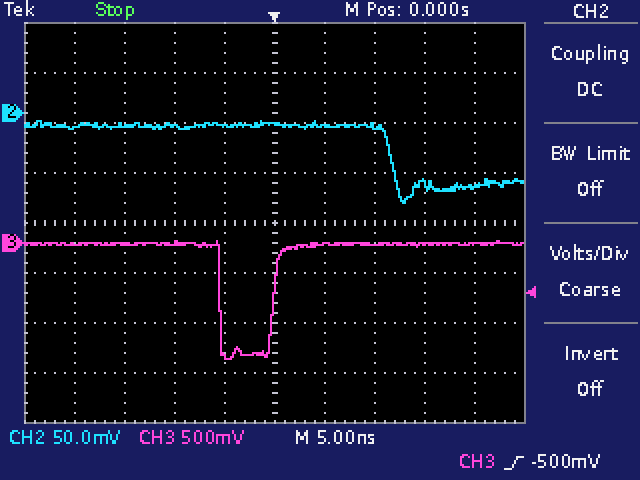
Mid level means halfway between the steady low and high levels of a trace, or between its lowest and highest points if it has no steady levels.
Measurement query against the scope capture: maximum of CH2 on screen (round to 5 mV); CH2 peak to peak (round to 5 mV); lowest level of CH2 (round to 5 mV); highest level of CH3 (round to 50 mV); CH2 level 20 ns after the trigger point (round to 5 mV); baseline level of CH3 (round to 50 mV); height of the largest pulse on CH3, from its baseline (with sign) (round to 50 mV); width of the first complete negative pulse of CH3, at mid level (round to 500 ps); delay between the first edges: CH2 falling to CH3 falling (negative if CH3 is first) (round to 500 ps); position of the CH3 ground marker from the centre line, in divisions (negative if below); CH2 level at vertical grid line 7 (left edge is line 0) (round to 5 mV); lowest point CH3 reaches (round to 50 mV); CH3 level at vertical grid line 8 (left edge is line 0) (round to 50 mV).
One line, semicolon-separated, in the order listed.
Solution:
-10 mV; 80 mV; -90 mV; 0 mV; -75 mV; 0 mV; -1.15 V; 5.5 ns; -17.0 ns; -0.4 div; -15 mV; -1.15 V; 0 mV
